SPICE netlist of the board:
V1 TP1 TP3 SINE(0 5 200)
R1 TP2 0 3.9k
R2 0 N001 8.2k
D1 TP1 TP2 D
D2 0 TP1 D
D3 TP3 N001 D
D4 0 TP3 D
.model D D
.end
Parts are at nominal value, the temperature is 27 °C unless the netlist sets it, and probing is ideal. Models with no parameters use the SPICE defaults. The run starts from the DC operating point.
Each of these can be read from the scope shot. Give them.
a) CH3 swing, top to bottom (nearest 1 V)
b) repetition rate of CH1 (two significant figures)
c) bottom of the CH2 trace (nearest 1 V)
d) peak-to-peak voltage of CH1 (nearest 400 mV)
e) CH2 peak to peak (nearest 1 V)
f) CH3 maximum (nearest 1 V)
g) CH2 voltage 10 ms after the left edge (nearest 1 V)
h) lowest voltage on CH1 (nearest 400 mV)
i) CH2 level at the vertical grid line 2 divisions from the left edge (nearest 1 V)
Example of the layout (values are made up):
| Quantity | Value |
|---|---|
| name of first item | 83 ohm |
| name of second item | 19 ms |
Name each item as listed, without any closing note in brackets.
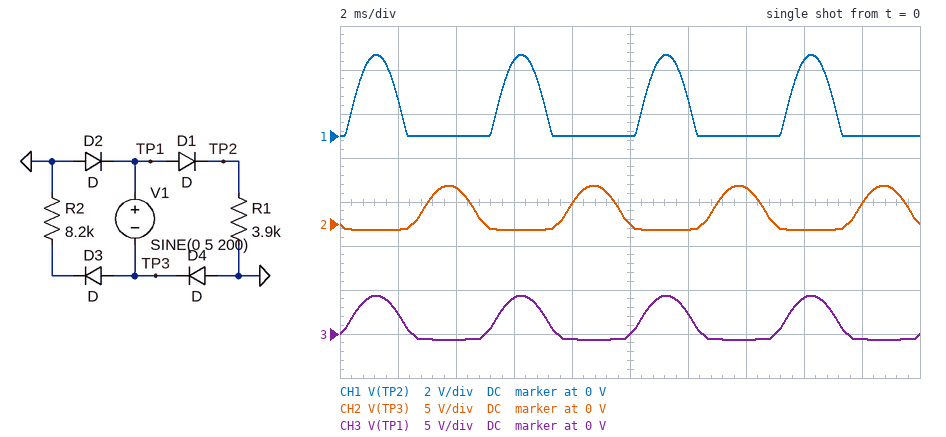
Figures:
| Quantity | Value |
|---|---|
| CH3 swing, top to bottom | 5 V |
| repetition rate of CH1 | 200 Hz |
| bottom of the CH2 trace | -1 V |
| peak-to-peak voltage of CH1 | 3.6 V |
| CH2 peak to peak | 5 V |
| CH3 maximum | 4 V |
| CH2 voltage 10 ms after the left edge | 0 V |
| lowest voltage on CH1 | 0 V |
| CH2 level at the vertical grid line 2 divisions from the left edge | 4 V |
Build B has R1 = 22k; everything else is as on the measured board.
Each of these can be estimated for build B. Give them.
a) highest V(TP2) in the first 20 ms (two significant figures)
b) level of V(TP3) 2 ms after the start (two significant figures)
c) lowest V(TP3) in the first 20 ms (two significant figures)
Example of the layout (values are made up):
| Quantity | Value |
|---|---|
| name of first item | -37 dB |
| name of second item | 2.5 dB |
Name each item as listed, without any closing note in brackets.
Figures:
| Quantity | Value |
|---|---|
| highest V(TP2) in the first 20 ms | 3.8 V |
| level of V(TP3) 2 ms after the start | -590 mV |
| lowest V(TP3) in the first 20 ms | -610 mV |
